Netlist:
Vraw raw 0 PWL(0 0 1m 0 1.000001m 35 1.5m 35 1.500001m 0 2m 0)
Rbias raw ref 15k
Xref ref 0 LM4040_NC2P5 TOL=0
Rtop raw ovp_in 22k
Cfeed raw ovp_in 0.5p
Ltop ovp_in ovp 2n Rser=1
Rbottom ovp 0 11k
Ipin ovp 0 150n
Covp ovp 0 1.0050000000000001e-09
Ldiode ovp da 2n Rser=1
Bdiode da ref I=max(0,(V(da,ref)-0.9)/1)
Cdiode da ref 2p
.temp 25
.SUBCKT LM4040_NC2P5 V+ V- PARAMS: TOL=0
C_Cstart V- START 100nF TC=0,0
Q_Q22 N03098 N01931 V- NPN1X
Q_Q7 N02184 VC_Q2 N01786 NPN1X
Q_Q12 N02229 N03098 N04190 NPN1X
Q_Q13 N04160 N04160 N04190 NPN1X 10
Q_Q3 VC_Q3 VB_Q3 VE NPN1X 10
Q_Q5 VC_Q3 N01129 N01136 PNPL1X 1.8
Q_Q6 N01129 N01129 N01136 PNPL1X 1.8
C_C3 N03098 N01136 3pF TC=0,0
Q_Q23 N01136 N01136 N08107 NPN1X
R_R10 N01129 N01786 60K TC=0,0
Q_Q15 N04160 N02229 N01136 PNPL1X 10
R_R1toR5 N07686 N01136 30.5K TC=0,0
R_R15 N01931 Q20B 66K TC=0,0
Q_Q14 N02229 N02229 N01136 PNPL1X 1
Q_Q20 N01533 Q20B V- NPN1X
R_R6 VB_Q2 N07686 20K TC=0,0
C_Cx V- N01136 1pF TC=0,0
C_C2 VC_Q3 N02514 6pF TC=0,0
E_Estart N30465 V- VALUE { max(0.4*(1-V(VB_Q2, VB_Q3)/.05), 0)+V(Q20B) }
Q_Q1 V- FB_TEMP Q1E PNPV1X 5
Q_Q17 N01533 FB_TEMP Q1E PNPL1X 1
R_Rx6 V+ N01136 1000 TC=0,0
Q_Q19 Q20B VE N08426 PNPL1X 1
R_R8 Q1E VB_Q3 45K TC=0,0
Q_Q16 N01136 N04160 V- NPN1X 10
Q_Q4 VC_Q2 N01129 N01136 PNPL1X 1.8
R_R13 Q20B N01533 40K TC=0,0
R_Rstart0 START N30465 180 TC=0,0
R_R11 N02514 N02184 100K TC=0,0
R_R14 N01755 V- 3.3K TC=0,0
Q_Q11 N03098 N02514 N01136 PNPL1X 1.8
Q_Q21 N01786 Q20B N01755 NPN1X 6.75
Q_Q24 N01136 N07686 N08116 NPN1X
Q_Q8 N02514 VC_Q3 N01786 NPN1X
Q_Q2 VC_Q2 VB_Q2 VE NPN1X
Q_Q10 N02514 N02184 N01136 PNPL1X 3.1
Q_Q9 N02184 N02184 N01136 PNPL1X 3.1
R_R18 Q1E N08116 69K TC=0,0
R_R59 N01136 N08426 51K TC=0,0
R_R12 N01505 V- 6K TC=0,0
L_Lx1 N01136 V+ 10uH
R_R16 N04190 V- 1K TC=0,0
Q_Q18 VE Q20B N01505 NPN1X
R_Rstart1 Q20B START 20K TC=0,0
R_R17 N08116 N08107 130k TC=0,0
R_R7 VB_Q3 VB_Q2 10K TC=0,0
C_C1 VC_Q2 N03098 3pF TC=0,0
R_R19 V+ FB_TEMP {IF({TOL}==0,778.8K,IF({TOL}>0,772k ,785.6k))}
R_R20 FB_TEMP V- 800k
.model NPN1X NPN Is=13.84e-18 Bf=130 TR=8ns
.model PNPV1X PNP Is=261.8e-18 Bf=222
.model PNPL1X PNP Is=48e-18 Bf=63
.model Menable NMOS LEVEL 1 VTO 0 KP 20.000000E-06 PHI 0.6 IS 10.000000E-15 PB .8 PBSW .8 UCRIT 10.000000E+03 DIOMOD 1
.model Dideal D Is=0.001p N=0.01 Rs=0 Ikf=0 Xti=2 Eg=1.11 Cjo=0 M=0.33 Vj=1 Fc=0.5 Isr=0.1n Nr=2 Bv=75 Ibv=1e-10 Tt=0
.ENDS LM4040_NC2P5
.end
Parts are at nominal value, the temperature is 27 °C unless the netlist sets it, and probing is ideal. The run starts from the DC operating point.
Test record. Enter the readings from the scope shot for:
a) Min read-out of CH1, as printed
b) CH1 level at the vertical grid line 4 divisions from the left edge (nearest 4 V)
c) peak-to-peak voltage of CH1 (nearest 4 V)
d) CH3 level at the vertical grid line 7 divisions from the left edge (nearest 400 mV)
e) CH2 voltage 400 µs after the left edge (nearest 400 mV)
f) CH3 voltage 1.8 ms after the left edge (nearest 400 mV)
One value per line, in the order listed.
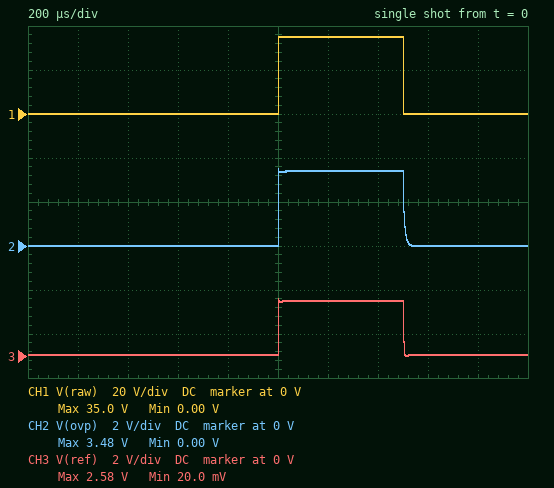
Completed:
0.00 V
0 V
36 V
2.4 V
0 V
0 V
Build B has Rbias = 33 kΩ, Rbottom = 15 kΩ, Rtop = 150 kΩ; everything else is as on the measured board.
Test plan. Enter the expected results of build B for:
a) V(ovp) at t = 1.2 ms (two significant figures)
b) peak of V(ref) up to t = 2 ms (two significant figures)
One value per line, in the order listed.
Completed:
3.2 V
2.5 V
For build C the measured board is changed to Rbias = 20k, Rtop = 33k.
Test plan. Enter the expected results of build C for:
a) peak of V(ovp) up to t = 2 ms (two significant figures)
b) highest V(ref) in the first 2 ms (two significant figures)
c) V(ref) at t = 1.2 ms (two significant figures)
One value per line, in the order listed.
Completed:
3.4 V
2.5 V
2.5 V
